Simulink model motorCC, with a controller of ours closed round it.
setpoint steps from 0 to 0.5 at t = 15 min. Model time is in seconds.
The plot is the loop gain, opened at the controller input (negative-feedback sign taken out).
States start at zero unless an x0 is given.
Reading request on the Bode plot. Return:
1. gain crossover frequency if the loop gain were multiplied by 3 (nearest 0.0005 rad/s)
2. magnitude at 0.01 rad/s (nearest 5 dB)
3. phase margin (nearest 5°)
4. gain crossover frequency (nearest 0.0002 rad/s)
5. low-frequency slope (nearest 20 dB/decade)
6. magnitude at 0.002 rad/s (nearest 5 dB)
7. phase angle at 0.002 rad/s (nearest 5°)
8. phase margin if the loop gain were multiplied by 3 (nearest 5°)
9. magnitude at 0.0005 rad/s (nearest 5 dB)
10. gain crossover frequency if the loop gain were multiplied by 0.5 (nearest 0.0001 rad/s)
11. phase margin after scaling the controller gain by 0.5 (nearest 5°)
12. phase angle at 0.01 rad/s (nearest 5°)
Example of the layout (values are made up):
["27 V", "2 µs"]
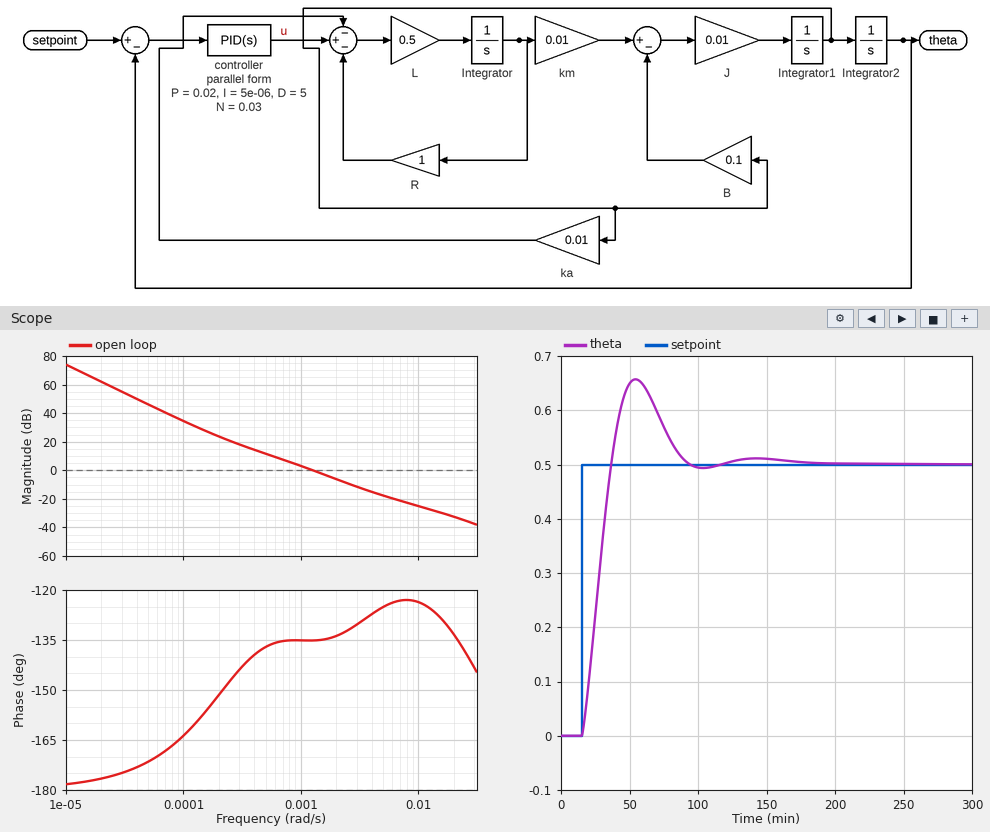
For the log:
["0.0025 rad/s", "-25 dB", "45°", "0.0012 rad/s", "-40 dB/decade", "-5 dB", "-135°", "50°", "10 dB", "0.0008 rad/s", "45°", "-125°"]
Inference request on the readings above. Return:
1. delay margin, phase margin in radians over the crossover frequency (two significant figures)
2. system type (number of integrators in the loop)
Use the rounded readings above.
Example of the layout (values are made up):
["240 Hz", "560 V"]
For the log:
["650 s", "2"]
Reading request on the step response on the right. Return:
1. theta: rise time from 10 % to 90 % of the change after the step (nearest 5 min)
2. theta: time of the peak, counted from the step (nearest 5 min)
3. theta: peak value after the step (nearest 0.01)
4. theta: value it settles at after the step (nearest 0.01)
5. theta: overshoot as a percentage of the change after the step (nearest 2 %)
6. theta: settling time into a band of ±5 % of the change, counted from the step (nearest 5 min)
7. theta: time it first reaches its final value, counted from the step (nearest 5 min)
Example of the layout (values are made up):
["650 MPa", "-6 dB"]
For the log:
["15 min", "40 min", "0.66", "0.50", "32 %", "70 min", "20 min"]
